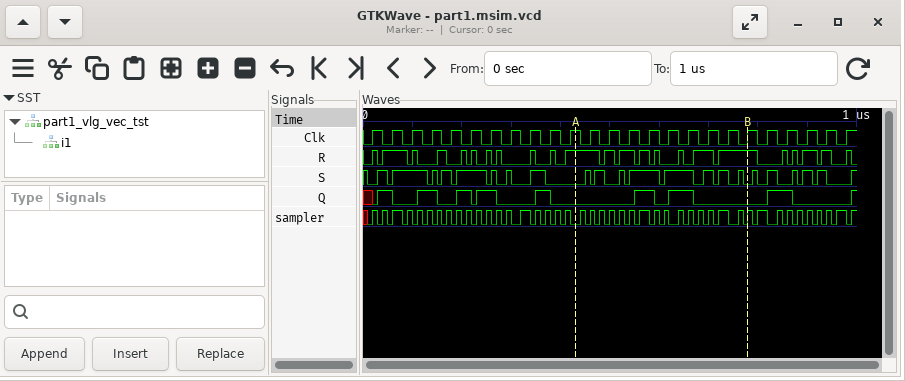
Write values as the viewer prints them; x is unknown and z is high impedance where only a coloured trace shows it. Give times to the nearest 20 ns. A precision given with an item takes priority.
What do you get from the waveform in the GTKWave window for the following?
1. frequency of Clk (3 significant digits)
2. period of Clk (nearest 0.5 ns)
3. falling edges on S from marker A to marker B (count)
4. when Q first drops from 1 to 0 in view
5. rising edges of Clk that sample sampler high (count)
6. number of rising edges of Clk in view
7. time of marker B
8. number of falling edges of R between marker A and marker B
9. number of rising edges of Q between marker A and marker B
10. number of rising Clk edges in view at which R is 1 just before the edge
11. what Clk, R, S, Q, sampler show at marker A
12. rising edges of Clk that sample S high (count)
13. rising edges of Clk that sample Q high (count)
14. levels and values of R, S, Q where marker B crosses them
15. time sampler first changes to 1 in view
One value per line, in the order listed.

25.0 MHz
40 ns
8
60 ns
14
25
780 ns
7
2
13
Clk=1, R=1, S=0, Q=0, sampler=0
12
8
R=1, S=0, Q=0
20 ns
